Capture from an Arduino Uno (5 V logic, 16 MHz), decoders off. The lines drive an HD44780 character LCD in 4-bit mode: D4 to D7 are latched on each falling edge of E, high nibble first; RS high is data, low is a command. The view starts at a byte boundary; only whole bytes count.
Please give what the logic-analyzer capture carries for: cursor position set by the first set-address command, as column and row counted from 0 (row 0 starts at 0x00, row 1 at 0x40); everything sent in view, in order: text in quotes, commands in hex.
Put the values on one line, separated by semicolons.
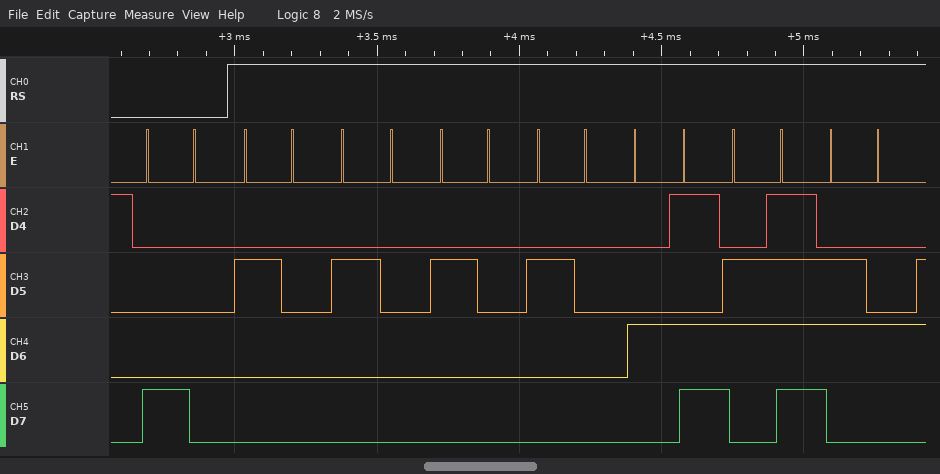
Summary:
column 0, row 0; 0x80 "    Mod"
